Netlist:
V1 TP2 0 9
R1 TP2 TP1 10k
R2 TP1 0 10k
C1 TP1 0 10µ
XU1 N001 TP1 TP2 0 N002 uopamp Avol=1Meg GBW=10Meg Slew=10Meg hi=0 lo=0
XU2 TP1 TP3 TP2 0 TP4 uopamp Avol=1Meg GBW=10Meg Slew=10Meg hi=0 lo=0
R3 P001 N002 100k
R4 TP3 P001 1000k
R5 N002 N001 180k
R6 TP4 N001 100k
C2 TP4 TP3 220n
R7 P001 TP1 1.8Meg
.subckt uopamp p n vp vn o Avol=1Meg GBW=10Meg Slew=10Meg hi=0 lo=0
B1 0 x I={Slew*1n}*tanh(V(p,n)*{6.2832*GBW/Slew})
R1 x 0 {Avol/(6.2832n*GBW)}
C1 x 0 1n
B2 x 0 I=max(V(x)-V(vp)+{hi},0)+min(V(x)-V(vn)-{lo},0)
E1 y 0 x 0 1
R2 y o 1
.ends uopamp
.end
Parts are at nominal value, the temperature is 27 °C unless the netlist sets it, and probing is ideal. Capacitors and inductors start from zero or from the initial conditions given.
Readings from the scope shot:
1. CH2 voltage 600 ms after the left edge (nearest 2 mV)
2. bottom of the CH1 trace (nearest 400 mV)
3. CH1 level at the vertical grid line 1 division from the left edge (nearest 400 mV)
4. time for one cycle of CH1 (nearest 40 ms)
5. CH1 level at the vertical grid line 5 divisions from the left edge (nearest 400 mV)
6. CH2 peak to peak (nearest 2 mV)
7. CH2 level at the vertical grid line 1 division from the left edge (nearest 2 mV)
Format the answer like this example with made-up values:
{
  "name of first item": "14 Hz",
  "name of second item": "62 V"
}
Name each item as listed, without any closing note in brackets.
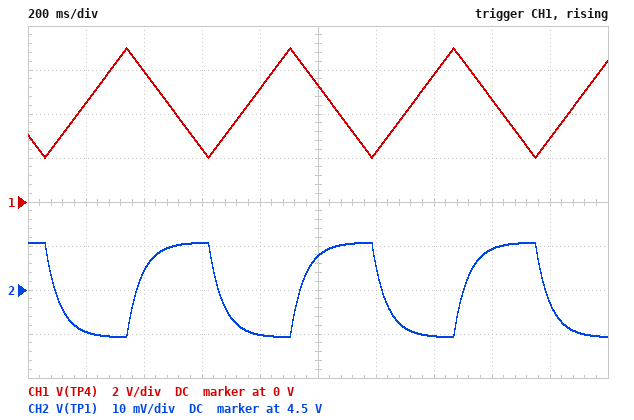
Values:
{
  "CH2 voltage 600 ms after the left edge": "4.510 V",
  "bottom of the CH1 trace": "2.0 V",
  "CH1 level at the vertical grid line 1 division from the left edge": "4.4 V",
  "time for one cycle of CH1": "560 ms",
  "CH1 level at the vertical grid line 5 divisions from the left edge": "5.2 V",
  "CH2 peak to peak": "22 mV",
  "CH2 level at the vertical grid line 1 division from the left edge": "4.490 V"
}
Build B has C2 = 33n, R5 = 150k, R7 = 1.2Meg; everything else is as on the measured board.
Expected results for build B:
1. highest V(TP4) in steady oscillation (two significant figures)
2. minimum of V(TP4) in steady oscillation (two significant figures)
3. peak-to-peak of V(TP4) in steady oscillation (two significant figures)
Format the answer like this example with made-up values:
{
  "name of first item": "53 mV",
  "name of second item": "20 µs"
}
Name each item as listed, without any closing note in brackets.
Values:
{
  "highest V(TP4) in steady oscillation": "7.5 V",
  "minimum of V(TP4) in steady oscillation": "1.5 V",
  "peak-to-peak of V(TP4) in steady oscillation": "6.0 V"
}
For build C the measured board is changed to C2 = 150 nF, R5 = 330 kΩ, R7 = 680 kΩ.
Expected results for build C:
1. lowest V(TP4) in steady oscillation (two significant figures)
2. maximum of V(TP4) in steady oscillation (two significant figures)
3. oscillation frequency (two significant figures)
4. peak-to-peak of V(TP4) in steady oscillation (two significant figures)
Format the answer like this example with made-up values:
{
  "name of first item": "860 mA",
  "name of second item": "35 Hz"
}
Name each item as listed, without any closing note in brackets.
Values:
{
  "lowest V(TP4) in steady oscillation": "3.2 V",
  "maximum of V(TP4) in steady oscillation": "5.8 V",
  "oscillation frequency": "4.4 Hz",
  "peak-to-peak of V(TP4) in steady oscillation": "2.7 V"
}
